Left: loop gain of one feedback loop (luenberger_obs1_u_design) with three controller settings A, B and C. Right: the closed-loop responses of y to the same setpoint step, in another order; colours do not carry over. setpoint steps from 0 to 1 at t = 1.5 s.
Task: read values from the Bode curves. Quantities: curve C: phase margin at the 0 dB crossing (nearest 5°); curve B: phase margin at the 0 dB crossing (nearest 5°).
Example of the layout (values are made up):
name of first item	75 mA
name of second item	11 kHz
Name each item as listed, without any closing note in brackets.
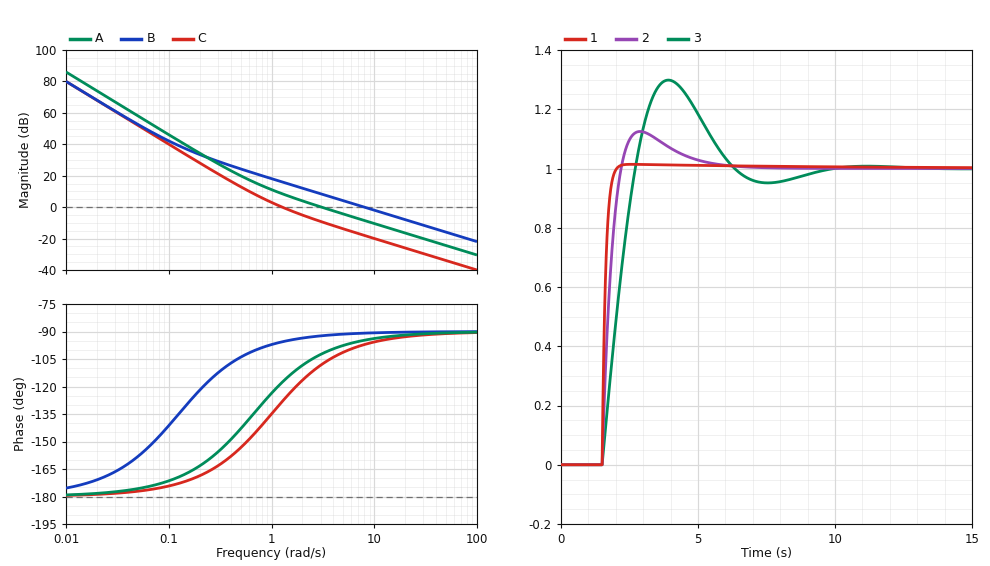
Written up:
curve C: phase margin at the 0 dB crossing	50°
curve B: phase margin at the 0 dB crossing	90°
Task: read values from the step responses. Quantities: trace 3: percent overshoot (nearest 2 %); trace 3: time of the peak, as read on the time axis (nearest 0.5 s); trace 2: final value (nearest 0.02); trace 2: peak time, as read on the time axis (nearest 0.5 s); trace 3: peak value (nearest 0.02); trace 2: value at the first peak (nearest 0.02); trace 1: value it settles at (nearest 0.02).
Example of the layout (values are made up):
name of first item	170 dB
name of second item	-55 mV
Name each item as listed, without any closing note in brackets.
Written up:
trace 3: percent overshoot	30 %
trace 3: time of the peak, as read on the time axis	4.0 s
trace 2: final value	1.00
trace 2: peak time, as read on the time axis	3.0 s
trace 3: peak value	1.30
trace 2: value at the first peak	1.12
trace 1: value it settles at	1.00
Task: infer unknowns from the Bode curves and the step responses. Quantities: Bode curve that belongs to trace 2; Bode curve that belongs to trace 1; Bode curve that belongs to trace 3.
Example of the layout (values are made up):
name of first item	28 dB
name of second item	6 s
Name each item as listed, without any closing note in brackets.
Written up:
Bode curve that belongs to trace 2	A
Bode curve that belongs to trace 1	B
Bode curve that belongs to trace 3	C
